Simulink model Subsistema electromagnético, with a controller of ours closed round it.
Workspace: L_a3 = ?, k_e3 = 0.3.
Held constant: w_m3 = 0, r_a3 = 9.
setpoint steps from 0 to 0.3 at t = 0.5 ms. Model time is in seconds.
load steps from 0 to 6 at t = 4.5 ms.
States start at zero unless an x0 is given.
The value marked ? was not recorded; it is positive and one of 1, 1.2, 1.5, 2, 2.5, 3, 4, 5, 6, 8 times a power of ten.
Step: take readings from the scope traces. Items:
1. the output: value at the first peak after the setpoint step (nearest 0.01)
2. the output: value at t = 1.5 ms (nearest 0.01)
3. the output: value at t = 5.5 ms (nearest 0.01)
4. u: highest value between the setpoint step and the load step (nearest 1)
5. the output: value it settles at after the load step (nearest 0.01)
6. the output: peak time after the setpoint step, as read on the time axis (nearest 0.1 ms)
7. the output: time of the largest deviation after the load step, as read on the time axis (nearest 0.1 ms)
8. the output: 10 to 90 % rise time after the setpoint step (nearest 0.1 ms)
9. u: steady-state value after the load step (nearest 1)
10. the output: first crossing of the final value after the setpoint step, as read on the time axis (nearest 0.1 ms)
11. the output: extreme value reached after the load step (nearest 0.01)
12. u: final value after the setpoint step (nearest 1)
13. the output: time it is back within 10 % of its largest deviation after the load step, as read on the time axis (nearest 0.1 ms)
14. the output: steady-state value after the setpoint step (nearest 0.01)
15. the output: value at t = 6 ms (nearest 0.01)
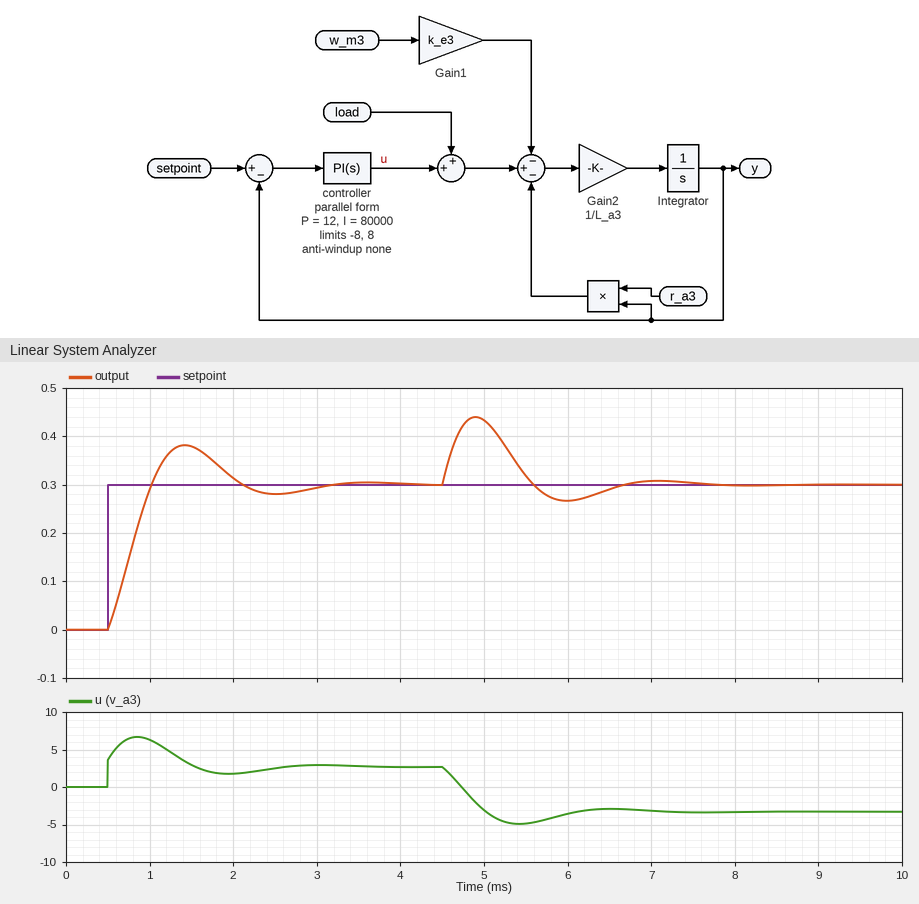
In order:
0.38
0.38
0.32
7
0.30
1.4 ms
4.9 ms
0.4 ms
-3
1.0 ms
0.44
3
6.4 ms
0.30
0.27
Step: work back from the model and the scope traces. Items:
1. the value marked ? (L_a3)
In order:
0.008
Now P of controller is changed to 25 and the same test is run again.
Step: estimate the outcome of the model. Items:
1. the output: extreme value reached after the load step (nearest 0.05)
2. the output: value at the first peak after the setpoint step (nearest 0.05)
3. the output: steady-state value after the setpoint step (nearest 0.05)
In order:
0.40
0.35
0.30
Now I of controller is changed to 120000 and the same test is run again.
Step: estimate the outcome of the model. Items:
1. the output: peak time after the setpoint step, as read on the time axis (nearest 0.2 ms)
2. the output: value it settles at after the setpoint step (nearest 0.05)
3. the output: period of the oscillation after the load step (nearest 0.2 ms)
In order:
1.2 ms
0.30
1.8 ms
